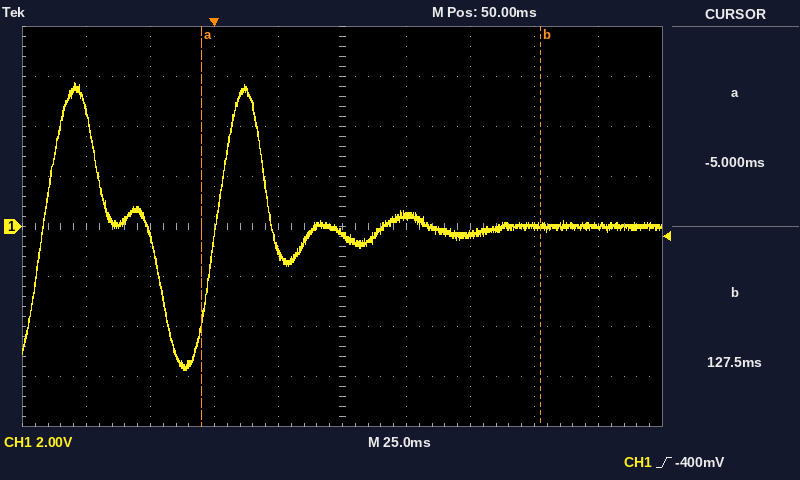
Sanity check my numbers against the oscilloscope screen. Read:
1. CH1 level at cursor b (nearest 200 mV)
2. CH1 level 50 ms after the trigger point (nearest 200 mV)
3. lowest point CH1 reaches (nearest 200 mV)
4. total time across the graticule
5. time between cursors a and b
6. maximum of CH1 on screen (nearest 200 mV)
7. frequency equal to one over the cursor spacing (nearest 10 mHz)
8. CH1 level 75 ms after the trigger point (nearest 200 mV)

0.0 V
-200 mV
-5.8 V
250 ms
132.5 ms
5.8 V
7.55 Hz
400 mV
